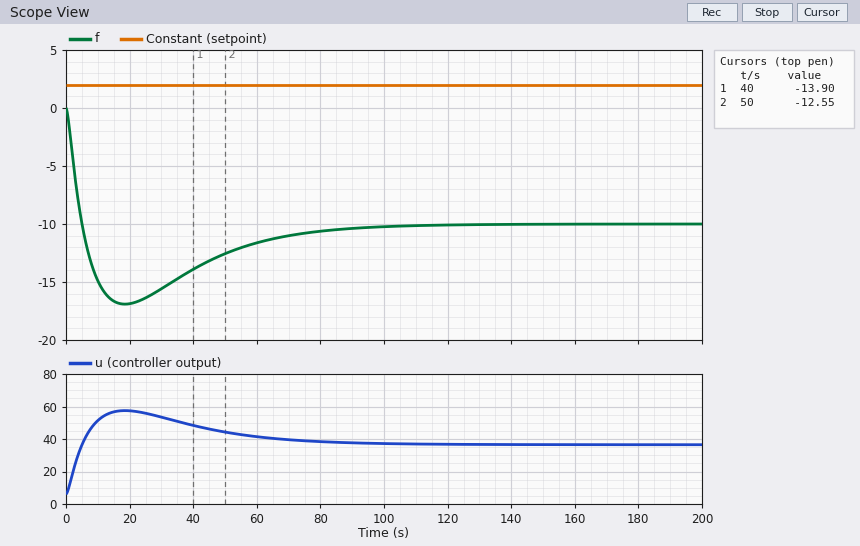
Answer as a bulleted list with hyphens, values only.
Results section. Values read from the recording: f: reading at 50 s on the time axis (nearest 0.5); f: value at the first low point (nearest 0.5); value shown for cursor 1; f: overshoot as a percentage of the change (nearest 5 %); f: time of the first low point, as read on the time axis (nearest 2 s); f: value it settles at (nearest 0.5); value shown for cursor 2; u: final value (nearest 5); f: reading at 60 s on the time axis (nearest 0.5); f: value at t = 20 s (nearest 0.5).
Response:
- -12.5
- -17.0
- -13.90
- 70 %
- 18 s
- -10.0
- -12.55
- 35
- -11.5
- -17.0
